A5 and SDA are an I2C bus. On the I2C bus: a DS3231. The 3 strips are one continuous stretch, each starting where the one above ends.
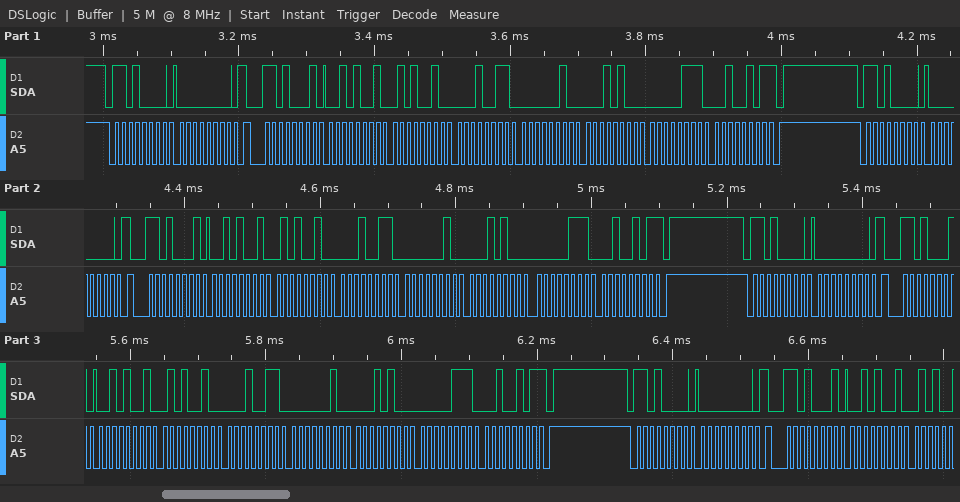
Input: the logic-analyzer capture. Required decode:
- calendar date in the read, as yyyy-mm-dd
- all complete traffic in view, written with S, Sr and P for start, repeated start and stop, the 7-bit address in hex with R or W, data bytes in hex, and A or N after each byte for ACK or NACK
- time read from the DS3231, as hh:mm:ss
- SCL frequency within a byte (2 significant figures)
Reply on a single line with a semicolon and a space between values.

2025-07-14; S 68W A 00 A Sr 68R A 29 A 52 A 13 A 02 A 14 A 07 A 25 N P S 68W A 00 A Sr 68R A 29 A 52 A 13 A 02 A 14 A 07 A 25 N P S 68W A 00 A Sr 68R A 29 A 52 A 13 A 02 A 14 A 07 A 25 N P S 68W A 00 A Sr 68R A 29 A; 13:52:29; 100 kHz
